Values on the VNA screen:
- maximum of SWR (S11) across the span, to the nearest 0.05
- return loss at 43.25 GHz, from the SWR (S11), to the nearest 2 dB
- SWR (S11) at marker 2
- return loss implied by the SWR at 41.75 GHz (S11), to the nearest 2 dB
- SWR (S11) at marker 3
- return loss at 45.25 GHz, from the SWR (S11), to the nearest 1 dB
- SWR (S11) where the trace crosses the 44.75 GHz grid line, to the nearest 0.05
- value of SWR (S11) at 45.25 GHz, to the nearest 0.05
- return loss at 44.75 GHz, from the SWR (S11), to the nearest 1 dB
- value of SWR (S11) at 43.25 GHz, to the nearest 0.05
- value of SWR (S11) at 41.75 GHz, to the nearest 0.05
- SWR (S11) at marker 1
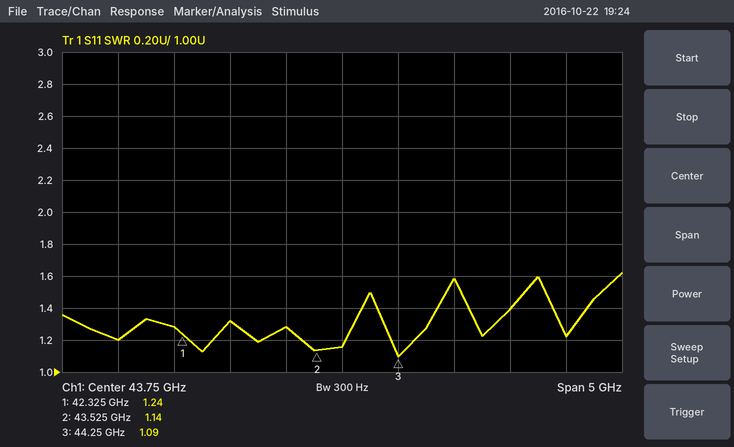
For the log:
1.60
18 dB
1.14
20 dB
1.09
16 dB
1.60
1.40
13 dB
1.30
1.20
1.24
